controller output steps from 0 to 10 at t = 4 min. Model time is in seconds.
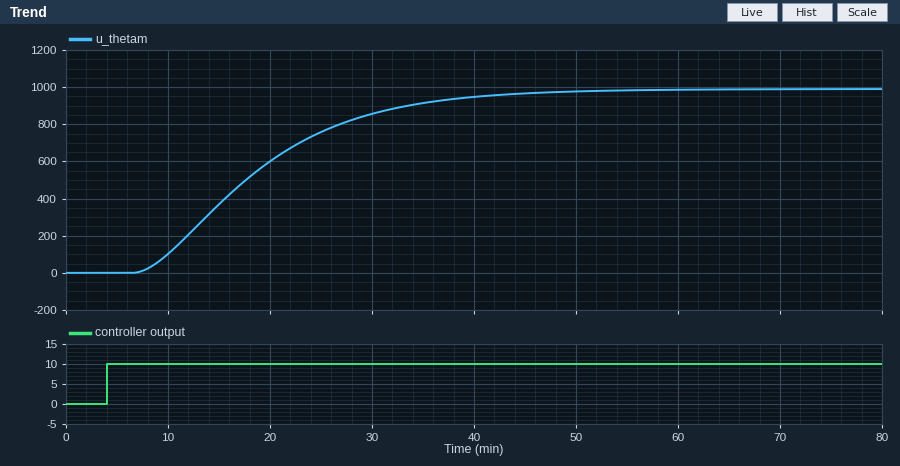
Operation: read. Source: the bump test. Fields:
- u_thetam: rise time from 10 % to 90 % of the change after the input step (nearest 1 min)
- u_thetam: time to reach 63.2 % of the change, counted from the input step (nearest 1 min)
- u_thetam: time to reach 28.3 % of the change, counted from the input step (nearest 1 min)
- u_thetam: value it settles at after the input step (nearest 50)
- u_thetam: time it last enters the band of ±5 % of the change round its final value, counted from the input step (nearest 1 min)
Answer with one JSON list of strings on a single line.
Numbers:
["23 min", "17 min", "9 min", "1000", "35 min"]
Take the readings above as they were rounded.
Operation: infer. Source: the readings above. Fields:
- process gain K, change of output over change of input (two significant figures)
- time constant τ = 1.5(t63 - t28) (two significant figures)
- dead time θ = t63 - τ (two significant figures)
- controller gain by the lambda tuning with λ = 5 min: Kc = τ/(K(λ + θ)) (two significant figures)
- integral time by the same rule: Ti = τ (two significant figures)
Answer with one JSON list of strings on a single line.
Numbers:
["100", "12 min", "5.0 min", "0.012", "12 min"]
